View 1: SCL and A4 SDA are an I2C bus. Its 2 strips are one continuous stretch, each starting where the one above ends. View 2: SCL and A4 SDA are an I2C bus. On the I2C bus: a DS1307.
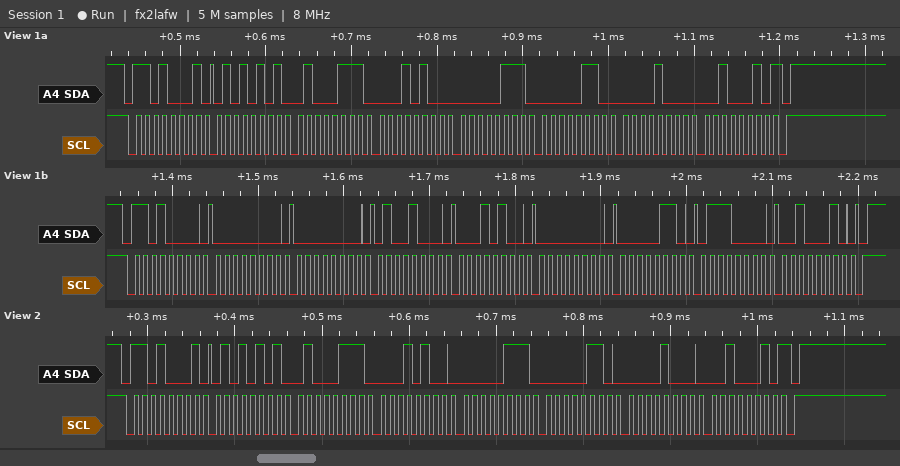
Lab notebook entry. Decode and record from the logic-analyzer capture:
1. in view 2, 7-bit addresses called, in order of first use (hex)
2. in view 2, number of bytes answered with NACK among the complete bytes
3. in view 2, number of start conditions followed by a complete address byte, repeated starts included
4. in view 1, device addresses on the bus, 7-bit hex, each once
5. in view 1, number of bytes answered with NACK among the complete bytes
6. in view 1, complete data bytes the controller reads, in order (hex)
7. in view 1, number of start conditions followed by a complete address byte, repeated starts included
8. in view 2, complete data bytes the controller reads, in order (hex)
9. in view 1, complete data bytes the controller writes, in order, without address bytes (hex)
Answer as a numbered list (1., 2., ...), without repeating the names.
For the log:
1. 0x68
2. 1
3. 1
4. 0x68
5. 1
6. 55 47 14 07 06 08 22
7. 2
8. 55 47 14 07 06 08 22
9. 00 00 48 14 00 06 70 22
